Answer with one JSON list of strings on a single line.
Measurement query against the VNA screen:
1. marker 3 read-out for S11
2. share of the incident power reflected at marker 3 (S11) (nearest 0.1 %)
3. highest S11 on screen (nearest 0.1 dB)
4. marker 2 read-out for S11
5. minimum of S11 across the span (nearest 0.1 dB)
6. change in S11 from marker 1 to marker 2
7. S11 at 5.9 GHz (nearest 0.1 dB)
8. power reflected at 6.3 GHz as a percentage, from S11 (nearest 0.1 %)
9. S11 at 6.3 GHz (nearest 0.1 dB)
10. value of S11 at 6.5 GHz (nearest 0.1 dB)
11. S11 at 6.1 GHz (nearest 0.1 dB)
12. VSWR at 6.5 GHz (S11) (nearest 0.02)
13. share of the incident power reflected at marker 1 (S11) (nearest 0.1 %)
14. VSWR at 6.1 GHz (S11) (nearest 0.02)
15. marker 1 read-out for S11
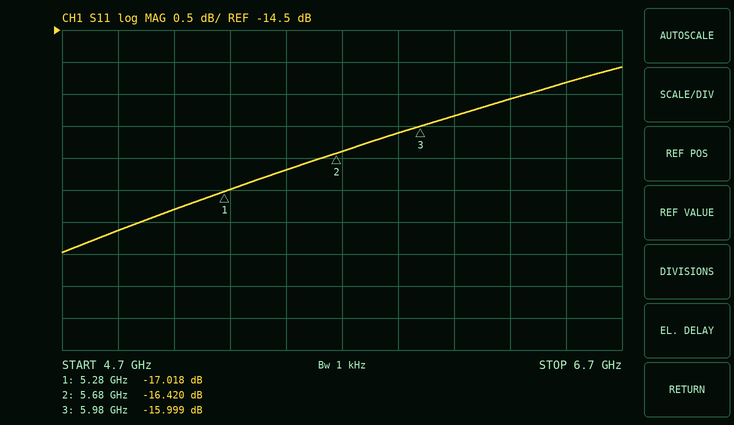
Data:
["-15.999 dB", "2.5 %", "-15.1 dB", "-16.420 dB", "-18.0 dB", "0.598 dB", "-16.1 dB", "2.8 %", "-15.6 dB", "-15.3 dB", "-15.8 dB", "1.42", "2.0 %", "1.38", "-17.018 dB"]
